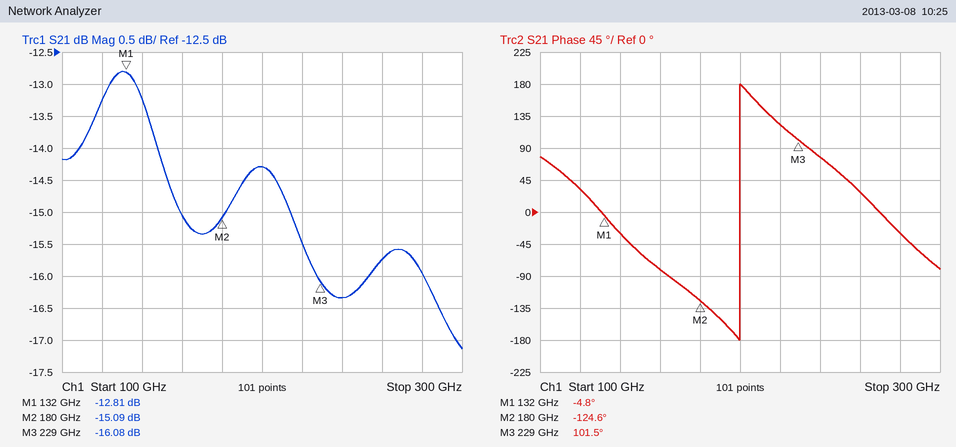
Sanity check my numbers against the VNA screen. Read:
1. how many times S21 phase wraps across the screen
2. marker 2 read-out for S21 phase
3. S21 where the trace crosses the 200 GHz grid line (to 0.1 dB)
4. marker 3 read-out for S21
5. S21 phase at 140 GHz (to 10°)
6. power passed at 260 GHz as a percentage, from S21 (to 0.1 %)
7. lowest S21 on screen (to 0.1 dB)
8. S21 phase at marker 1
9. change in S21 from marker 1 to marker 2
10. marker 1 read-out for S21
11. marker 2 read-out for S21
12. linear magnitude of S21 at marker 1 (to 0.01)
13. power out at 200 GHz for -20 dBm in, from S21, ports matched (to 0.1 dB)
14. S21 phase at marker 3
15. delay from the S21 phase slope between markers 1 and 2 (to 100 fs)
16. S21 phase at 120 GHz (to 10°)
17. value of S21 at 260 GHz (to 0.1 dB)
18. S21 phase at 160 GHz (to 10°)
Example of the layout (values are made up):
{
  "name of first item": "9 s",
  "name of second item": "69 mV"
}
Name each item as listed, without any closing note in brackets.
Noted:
{
  "how many times S21 phase wraps across the screen": "1",
  "marker 2 read-out for S21 phase": "-124.6°",
  "S21 where the trace crosses the 200 GHz grid line": "-14.3 dB",
  "marker 3 read-out for S21": "-16.08 dB",
  "S21 phase at 140 GHz": "-30°",
  "power passed at 260 GHz as a percentage, from S21": "2.7 %",
  "lowest S21 on screen": "-17.1 dB",
  "S21 phase at marker 1": "-4.8°",
  "change in S21 from marker 1 to marker 2": "-2.28 dB",
  "marker 1 read-out for S21": "-12.81 dB",
  "marker 2 read-out for S21": "-15.09 dB",
  "linear magnitude of S21 at marker 1": "0.23",
  "power out at 200 GHz for -20 dBm in, from S21, ports matched": "-34.3 dBm",
  "S21 phase at marker 3": "101.5°",
  "delay from the S21 phase slope between markers 1 and 2": "6.9 ps",
  "S21 phase at 120 GHz": "30°",
  "value of S21 at 260 GHz": "-15.7 dB",
  "S21 phase at 160 GHz": "-80°"
}
